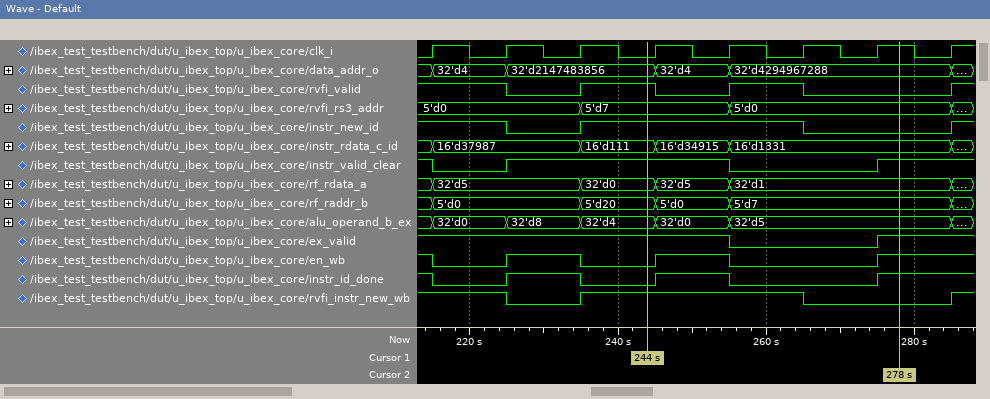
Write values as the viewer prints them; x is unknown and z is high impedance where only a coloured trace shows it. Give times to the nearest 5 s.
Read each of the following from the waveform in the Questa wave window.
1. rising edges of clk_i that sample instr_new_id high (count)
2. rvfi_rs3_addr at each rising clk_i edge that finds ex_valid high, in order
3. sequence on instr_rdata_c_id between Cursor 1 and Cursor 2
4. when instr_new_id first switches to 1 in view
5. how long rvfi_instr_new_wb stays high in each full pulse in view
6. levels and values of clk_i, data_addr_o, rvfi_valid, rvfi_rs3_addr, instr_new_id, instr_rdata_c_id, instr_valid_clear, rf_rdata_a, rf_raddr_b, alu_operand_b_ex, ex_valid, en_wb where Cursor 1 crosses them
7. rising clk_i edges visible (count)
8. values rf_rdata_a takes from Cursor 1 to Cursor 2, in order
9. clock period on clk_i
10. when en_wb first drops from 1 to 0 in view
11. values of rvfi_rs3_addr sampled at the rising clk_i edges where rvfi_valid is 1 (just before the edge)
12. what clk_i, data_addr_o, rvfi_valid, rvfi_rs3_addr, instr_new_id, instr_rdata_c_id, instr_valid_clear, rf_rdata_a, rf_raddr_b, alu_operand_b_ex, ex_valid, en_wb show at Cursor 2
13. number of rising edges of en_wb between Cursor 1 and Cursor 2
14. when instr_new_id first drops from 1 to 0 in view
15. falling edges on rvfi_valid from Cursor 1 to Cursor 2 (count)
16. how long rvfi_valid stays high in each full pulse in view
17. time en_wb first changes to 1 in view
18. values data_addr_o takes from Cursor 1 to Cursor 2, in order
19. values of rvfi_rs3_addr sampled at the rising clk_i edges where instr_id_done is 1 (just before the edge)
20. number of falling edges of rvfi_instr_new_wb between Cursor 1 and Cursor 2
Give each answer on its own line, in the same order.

5
5'd0, 5'd0, 5'd0, 5'd7, 5'd7, 5'd0
16'd111, 16'd34915, 16'd1331
235 s
30 s
clk_i=0, data_addr_o=32'd2147483856, rvfi_valid=1, rvfi_rs3_addr=5'd7, instr_new_id=1, instr_rdata_c_id=16'd111, instr_valid_clear=1, rf_rdata_a=32'd0, rf_raddr_b=5'd20, alu_operand_b_ex=32'd4, ex_valid=1, en_wb=0
8
32'd0, 32'd5, 32'd1
10 s
215 s
5'd0, 5'd0, 5'd7, 5'd0
clk_i=1, data_addr_o=32'd4294967288, rvfi_valid=0, rvfi_rs3_addr=5'd0, instr_new_id=0, instr_rdata_c_id=16'd1331, instr_valid_clear=1, rf_rdata_a=32'd1, rf_raddr_b=5'd7, alu_operand_b_ex=32'd5, ex_valid=1, en_wb=1
2
225 s
2
10 s, 10 s
225 s
32'd2147483856, 32'd4, 32'd4294967288
5'd0, 5'd0, 5'd7, 5'd0
1
